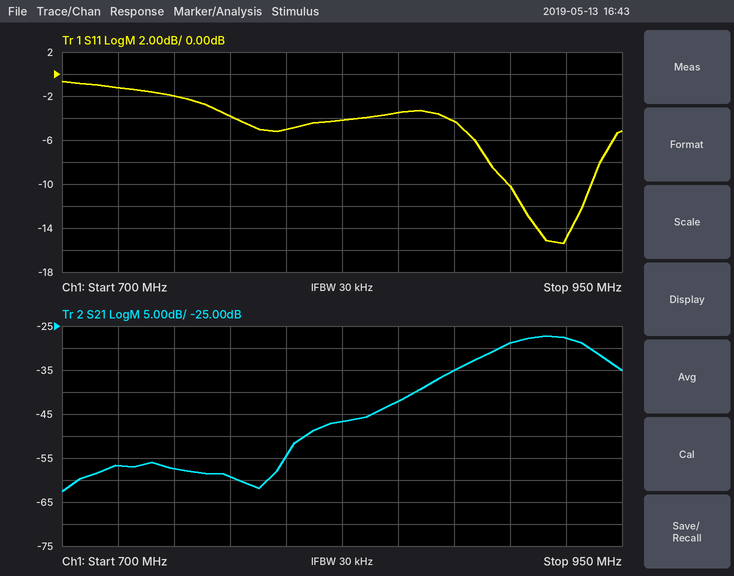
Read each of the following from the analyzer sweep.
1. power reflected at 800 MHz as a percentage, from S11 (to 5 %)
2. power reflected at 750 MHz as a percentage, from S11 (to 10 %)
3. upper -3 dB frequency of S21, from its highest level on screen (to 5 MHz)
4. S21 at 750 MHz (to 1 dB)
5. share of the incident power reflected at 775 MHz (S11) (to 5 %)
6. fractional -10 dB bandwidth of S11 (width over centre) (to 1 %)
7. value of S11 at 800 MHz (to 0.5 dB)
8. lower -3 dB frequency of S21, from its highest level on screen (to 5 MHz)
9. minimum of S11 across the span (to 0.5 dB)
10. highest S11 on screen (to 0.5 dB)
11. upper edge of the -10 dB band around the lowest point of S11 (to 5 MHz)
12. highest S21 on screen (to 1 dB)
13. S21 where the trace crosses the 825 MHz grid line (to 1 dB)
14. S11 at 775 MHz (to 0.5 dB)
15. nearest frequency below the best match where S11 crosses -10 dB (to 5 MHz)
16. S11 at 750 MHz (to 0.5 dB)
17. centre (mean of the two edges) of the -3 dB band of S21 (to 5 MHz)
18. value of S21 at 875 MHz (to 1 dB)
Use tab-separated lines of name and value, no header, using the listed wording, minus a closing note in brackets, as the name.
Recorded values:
power reflected at 800 MHz as a percentage, from S11	30 %
power reflected at 750 MHz as a percentage, from S11	60 %
upper -3 dB frequency of S21, from its highest level on screen	935 MHz
S21 at 750 MHz	-57 dB
share of the incident power reflected at 775 MHz (S11)	40 %
fractional -10 dB bandwidth of S11 (width over centre)	4 %
value of S11 at 800 MHz	-5.0 dB
lower -3 dB frequency of S21, from its highest level on screen	895 MHz
minimum of S11 across the span	-15.5 dB
highest S11 on screen	-0.5 dB
upper edge of the -10 dB band around the lowest point of S11	935 MHz
highest S21 on screen	-27 dB
S21 where the trace crosses the 825 MHz grid line	-47 dB
S11 at 775 MHz	-4.0 dB
nearest frequency below the best match where S11 crosses -10 dB	900 MHz
S11 at 750 MHz	-2.0 dB
centre (mean of the two edges) of the -3 dB band of S21	915 MHz
value of S21 at 875 MHz	-35 dB
